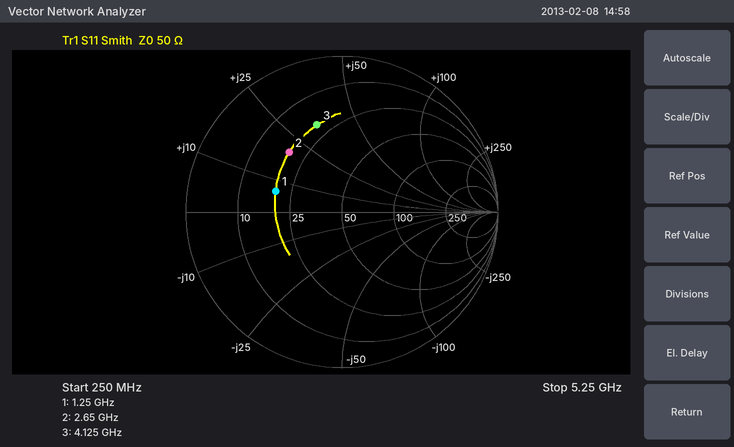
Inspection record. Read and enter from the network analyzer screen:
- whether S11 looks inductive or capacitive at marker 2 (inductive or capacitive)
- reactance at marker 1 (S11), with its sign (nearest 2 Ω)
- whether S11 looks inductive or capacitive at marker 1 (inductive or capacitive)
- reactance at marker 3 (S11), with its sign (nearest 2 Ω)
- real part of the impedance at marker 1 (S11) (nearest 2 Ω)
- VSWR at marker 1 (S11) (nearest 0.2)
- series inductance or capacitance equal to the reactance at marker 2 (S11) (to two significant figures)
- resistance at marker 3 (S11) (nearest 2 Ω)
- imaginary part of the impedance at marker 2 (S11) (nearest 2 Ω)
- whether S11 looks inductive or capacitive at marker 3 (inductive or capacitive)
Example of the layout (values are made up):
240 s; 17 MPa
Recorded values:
inductive; +6 Ω; inductive; +34 Ω; 20 Ω; 2.6; 1.2 nH; 20 Ω; +20 Ω; inductive
